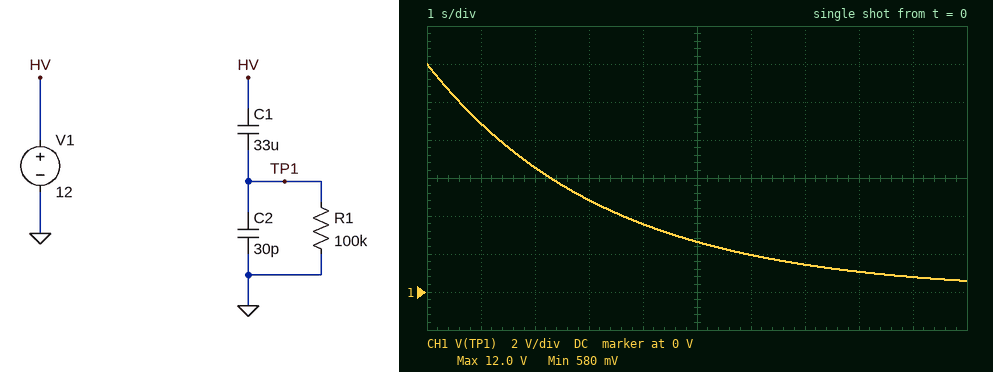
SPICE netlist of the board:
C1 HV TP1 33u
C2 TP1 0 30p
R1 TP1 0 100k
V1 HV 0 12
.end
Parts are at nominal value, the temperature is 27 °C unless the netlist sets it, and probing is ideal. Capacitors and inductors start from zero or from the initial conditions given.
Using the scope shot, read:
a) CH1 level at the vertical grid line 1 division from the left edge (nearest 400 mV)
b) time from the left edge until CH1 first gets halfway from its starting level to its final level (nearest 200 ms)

8.8 V
2.2 s
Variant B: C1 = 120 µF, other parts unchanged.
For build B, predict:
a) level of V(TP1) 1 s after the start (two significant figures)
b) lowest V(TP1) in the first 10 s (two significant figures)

11 V
5.2 V
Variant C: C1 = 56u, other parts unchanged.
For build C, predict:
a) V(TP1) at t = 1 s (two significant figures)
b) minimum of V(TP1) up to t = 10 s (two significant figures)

10 V
2.0 V
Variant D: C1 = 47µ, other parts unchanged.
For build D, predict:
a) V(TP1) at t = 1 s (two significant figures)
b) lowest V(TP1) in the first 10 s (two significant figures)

9.7 V
1.4 V
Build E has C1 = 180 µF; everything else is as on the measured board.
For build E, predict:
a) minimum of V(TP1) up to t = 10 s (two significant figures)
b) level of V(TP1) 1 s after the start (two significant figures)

6.9 V
11 V
